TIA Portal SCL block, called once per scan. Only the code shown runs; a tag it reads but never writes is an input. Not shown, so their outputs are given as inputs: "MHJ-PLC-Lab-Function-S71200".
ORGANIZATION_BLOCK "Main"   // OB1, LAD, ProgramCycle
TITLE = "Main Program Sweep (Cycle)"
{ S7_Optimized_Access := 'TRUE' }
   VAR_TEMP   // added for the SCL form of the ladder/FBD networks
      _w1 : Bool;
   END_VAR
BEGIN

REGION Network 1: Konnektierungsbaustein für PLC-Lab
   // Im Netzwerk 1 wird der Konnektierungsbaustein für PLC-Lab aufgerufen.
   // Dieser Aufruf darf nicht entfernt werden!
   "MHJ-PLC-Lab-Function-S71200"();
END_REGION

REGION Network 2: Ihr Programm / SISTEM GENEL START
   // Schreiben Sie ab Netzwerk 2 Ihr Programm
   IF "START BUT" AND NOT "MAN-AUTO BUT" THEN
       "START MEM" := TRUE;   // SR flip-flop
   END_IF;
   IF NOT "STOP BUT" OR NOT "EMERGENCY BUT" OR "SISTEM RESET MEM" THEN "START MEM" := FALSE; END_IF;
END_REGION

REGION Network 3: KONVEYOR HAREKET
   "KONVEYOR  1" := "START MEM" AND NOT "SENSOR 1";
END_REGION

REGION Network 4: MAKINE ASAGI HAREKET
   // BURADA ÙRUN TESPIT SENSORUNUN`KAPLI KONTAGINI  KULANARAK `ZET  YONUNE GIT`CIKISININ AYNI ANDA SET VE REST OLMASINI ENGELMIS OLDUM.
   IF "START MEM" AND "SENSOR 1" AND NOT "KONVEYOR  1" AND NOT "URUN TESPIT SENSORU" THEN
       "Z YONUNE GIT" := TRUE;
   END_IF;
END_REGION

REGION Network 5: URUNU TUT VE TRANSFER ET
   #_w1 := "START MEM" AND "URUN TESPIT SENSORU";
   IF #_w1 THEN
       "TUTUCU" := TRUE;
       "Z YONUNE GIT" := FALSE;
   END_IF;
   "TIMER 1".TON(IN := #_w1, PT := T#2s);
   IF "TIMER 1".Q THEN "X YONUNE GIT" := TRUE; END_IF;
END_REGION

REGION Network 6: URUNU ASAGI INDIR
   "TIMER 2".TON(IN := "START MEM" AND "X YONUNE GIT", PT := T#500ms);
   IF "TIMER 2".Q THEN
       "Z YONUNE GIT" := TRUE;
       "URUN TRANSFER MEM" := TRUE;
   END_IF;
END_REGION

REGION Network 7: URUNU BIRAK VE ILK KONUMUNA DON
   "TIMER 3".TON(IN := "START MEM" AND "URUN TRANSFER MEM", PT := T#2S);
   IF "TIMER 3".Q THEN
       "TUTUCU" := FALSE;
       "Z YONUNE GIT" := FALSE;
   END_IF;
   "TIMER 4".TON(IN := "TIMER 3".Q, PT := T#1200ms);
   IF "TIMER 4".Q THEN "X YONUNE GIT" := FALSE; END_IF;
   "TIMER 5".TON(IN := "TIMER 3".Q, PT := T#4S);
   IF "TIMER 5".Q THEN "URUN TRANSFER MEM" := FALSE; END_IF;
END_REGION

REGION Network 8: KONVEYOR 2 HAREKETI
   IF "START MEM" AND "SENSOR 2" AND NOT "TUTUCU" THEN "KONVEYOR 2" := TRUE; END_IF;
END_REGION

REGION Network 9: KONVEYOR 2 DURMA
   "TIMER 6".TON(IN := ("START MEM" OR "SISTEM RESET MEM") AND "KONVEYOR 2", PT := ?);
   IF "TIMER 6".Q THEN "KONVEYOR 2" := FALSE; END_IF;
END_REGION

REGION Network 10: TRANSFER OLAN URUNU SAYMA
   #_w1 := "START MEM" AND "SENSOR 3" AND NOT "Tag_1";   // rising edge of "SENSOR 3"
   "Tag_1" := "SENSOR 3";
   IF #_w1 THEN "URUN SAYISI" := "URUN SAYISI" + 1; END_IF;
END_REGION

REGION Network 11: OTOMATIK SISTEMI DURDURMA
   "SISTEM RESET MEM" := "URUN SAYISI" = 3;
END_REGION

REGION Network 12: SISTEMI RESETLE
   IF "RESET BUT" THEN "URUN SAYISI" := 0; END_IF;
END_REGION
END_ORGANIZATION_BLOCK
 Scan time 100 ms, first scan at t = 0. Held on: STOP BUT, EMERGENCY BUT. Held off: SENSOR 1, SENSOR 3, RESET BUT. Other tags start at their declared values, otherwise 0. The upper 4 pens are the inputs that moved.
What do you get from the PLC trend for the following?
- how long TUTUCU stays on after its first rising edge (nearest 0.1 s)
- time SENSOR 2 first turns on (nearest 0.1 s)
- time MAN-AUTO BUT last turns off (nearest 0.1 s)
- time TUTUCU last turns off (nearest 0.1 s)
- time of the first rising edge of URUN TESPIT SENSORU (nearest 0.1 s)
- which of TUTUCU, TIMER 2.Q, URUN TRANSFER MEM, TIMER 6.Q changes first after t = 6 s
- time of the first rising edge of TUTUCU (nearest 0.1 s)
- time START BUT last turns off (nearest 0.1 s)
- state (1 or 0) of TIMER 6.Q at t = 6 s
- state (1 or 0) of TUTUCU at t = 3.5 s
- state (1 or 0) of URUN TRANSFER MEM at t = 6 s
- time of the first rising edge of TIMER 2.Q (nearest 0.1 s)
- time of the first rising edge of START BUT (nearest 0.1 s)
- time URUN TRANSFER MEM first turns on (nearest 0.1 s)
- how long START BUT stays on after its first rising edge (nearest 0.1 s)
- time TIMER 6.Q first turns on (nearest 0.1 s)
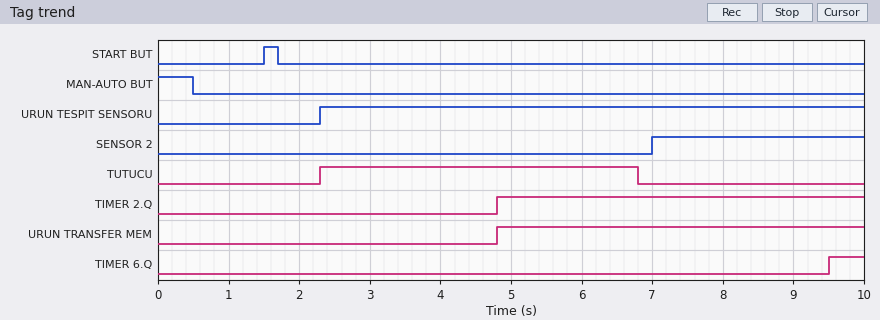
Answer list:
4.5 s
7.0 s
0.5 s
6.8 s
2.3 s
TUTUCU
2.3 s
1.7 s
0
1
1
4.8 s
1.5 s
4.8 s
0.2 s
9.5 s
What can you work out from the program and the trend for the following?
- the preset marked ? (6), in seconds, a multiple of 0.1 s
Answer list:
2.5 s
